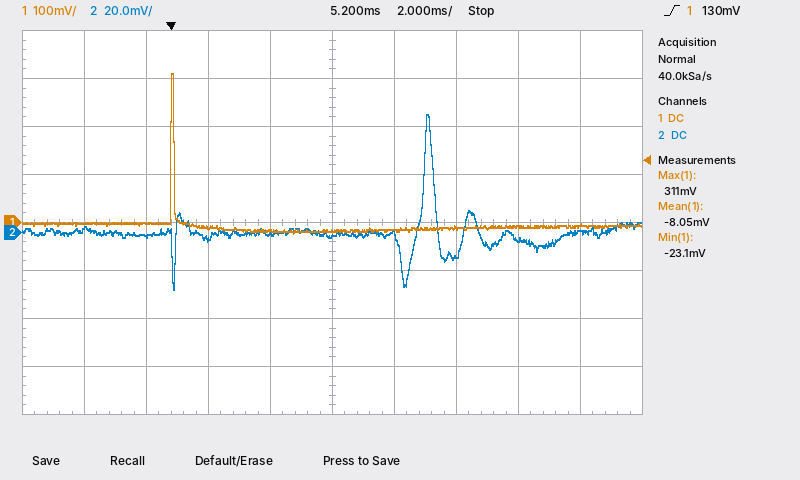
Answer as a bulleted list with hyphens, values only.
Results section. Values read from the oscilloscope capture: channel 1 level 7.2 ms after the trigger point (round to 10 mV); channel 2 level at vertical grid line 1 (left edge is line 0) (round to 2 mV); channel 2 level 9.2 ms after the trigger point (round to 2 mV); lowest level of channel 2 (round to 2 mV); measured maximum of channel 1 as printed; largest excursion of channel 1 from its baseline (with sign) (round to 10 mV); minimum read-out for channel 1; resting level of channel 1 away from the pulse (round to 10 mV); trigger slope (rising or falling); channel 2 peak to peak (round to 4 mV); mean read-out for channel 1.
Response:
- -20 mV
- 2 mV
- -10 mV
- -24 mV
- 311 mV
- +320 mV
- -23.1 mV
- -10 mV
- rising
- 72 mV
- -8.05 mV
